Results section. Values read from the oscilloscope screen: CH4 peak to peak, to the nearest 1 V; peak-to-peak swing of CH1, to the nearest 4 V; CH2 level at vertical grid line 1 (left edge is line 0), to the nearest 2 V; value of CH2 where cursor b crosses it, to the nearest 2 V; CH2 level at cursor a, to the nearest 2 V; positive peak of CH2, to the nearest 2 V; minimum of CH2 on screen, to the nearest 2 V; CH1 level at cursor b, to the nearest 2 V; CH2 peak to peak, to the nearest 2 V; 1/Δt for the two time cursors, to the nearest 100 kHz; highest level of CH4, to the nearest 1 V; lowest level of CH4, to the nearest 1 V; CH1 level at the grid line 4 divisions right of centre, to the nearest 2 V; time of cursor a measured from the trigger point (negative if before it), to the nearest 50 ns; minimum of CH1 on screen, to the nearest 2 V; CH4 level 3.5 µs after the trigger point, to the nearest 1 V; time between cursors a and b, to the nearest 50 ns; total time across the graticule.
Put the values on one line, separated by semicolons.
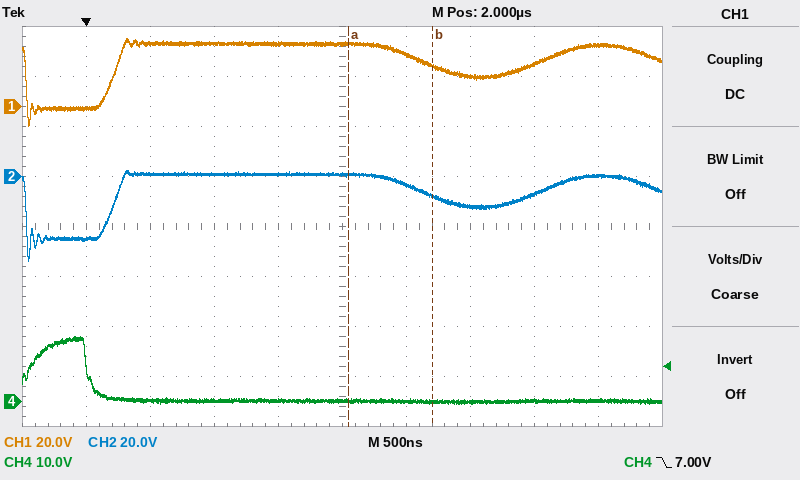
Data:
14 V; 36 V; -26 V; -8 V; 0 V; 2 V; -34 V; 16 V; 36 V; 1.5 MHz; 13 V; -1 V; 24 V; +2.05 µs; -8 V; 0 V; 650 ns; 5 µs
